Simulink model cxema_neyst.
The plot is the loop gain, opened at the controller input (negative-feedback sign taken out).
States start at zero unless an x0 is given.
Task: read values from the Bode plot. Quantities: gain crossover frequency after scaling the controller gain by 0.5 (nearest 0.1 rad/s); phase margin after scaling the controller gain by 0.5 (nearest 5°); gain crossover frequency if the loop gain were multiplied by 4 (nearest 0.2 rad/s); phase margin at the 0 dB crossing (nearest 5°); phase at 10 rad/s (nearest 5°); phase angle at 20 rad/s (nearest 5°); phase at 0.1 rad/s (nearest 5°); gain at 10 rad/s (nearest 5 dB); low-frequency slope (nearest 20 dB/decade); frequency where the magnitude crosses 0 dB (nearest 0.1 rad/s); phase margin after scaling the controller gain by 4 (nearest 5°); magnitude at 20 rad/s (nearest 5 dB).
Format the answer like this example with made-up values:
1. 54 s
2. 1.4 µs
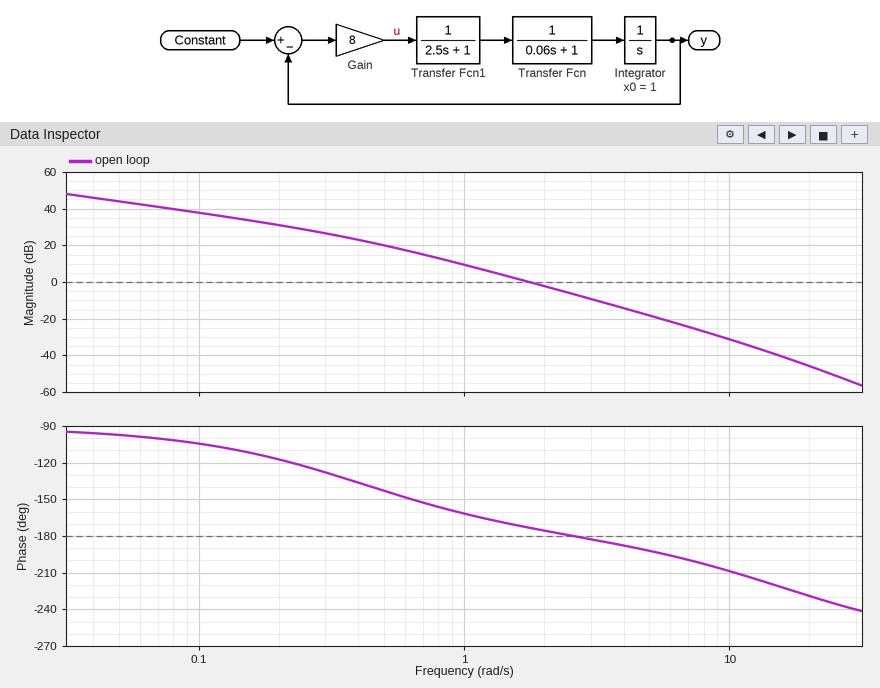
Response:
1. 1.2 rad/s
2. 15°
3. 3.6 rad/s
4. 5°
5. -210°
6. -230°
7. -105°
8. -30 dB
9. -20 dB/decade
10. 1.8 rad/s
11. -5°
12. -45 dB
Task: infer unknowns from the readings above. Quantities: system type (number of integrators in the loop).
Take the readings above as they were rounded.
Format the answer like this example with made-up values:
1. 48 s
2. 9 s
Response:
1. 1
